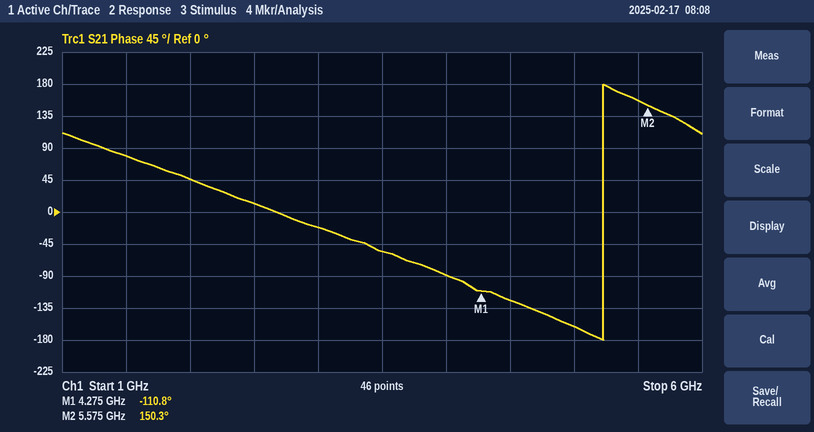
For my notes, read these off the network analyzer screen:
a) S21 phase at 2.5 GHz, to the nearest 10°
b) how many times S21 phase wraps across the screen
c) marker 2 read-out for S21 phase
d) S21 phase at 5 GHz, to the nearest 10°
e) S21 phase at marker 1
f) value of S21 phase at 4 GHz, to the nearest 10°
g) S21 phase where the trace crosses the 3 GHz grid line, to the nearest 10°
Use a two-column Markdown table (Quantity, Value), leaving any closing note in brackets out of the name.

| Quantity | Value |
|---|---|
| S21 phase at 2.5 GHz, to the nearest 10° | 10° |
| how many times S21 phase wraps across the screen | 1 |
| marker 2 read-out for S21 phase | 150.3° |
| S21 phase at 5 GHz, to the nearest 10° | -160° |
| S21 phase at marker 1 | -110.8° |
| value of S21 phase at 4 GHz, to the nearest 10° | -90° |
| S21 phase where the trace crosses the 3 GHz grid line, to the nearest 10° | -20° |
